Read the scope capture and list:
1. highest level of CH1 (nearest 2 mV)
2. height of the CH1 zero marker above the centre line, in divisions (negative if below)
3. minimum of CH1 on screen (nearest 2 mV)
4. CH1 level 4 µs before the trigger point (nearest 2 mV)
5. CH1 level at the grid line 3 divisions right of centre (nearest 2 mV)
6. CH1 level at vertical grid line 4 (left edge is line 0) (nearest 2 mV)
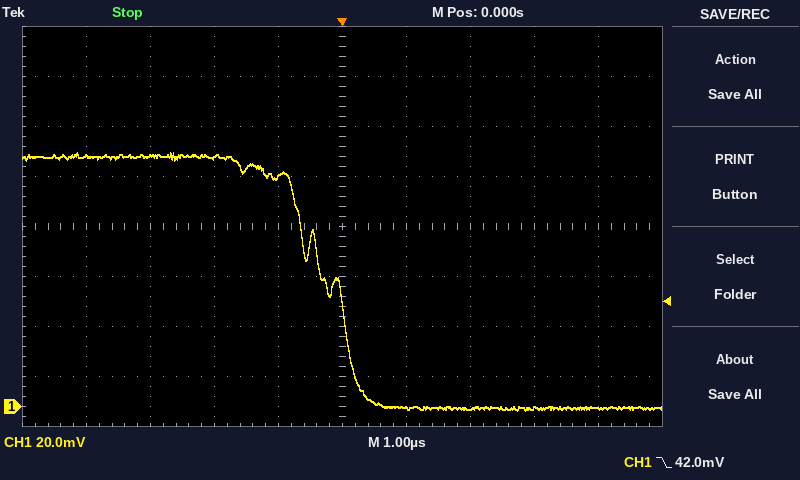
102 mV
-3.6 div
-2 mV
100 mV
0 mV
92 mV
